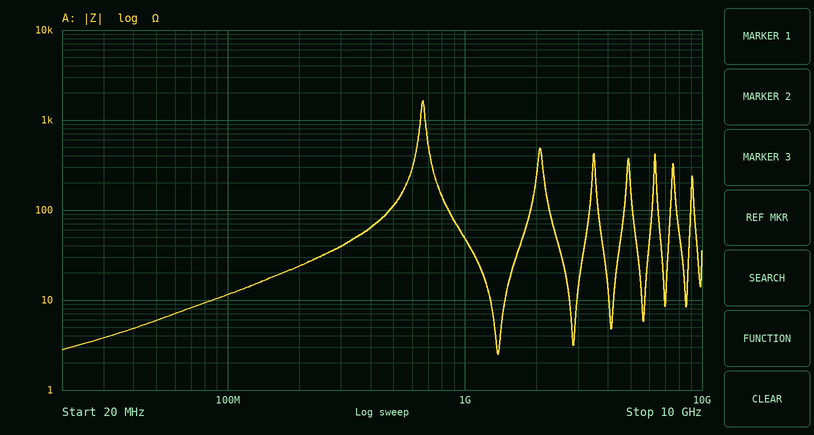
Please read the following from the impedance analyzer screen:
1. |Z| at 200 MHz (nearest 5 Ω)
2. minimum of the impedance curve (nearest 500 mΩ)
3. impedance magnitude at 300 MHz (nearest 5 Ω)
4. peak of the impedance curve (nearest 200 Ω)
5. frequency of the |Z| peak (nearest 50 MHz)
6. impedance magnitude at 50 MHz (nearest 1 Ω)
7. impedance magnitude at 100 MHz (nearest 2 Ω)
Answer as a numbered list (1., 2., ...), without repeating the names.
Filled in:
1. 25 Ω
2. 2.5 Ω
3. 40 Ω
4. 1.6 kΩ
5. 650 MHz
6. 6 Ω
7. 12 Ω
